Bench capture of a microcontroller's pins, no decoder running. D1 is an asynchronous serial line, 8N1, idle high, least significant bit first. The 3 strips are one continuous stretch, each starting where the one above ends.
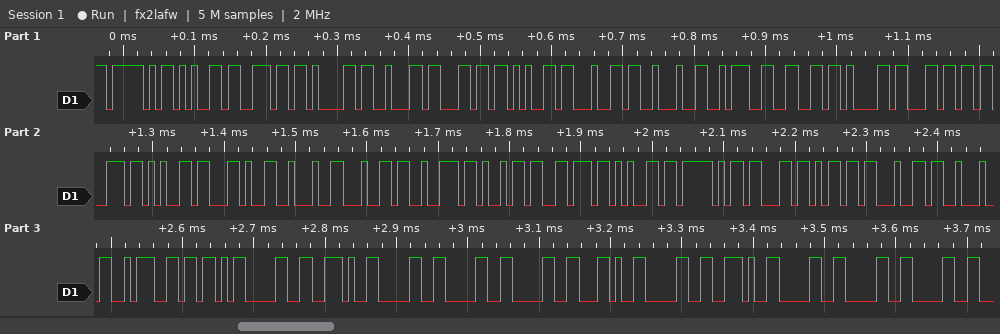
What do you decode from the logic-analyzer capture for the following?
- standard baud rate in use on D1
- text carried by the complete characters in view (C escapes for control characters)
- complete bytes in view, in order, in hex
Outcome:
115200 baud
"_enabled\":false,\"drive_cmd\":[0.000,0.000"
0x5F 0x65 0x6E 0x61 0x62 0x6C 0x65 0x64 0x22 0x3A 0x66 0x61 0x6C 0x73 0x65 0x2C 0x22 0x64 0x72 0x69 0x76 0x65 0x5F 0x63 0x6D 0x64 0x22 0x3A 0x5B 0x30 0x2E 0x30 0x30 0x30 0x2C 0x30 0x2E 0x30 0x30 0x30
